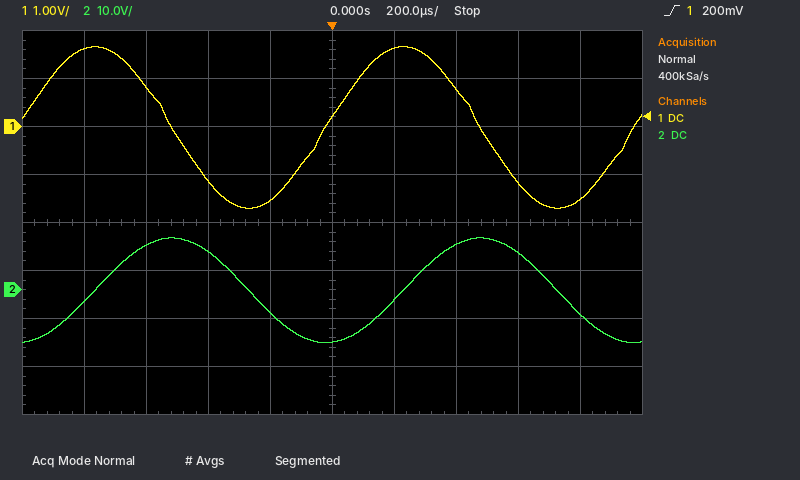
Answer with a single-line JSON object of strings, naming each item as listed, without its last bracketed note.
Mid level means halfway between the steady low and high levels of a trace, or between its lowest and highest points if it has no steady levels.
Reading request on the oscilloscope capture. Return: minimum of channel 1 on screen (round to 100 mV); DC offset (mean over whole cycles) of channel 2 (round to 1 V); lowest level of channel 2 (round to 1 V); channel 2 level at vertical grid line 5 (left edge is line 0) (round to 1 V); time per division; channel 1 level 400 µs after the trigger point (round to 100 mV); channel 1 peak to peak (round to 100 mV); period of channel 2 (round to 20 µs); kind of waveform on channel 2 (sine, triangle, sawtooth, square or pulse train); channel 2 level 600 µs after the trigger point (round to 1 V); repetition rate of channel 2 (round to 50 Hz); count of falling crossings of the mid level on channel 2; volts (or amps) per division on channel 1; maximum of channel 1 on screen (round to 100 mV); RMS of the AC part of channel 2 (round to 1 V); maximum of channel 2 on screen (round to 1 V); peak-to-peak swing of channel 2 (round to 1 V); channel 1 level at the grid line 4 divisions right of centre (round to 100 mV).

{"minimum of channel 1 on screen": "-1.7 V", "DC offset (mean over whole cycles) of channel 2": "0 V", "lowest level of channel 2": "-11 V", "channel 2 level at vertical grid line 5 (left edge is line 0)": "-11 V", "time per division": "200 µs", "channel 1 level 400 µs after the trigger point": "800 mV", "channel 1 peak to peak": "3.4 V", "period of channel 2": "1.00 ms", "kind of waveform on channel 2": "sine", "channel 2 level 600 µs after the trigger point": "8 V", "repetition rate of channel 2": "1.00 kHz", "count of falling crossings of the mid level on channel 2": "2", "volts (or amps) per division on channel 1": "1 V", "maximum of channel 1 on screen": "1.7 V", "RMS of the AC part of channel 2": "8 V", "maximum of channel 2 on screen": "11 V", "peak-to-peak swing of channel 2": "22 V", "channel 1 level at the grid line 4 divisions right of centre": "-1.5 V"}
